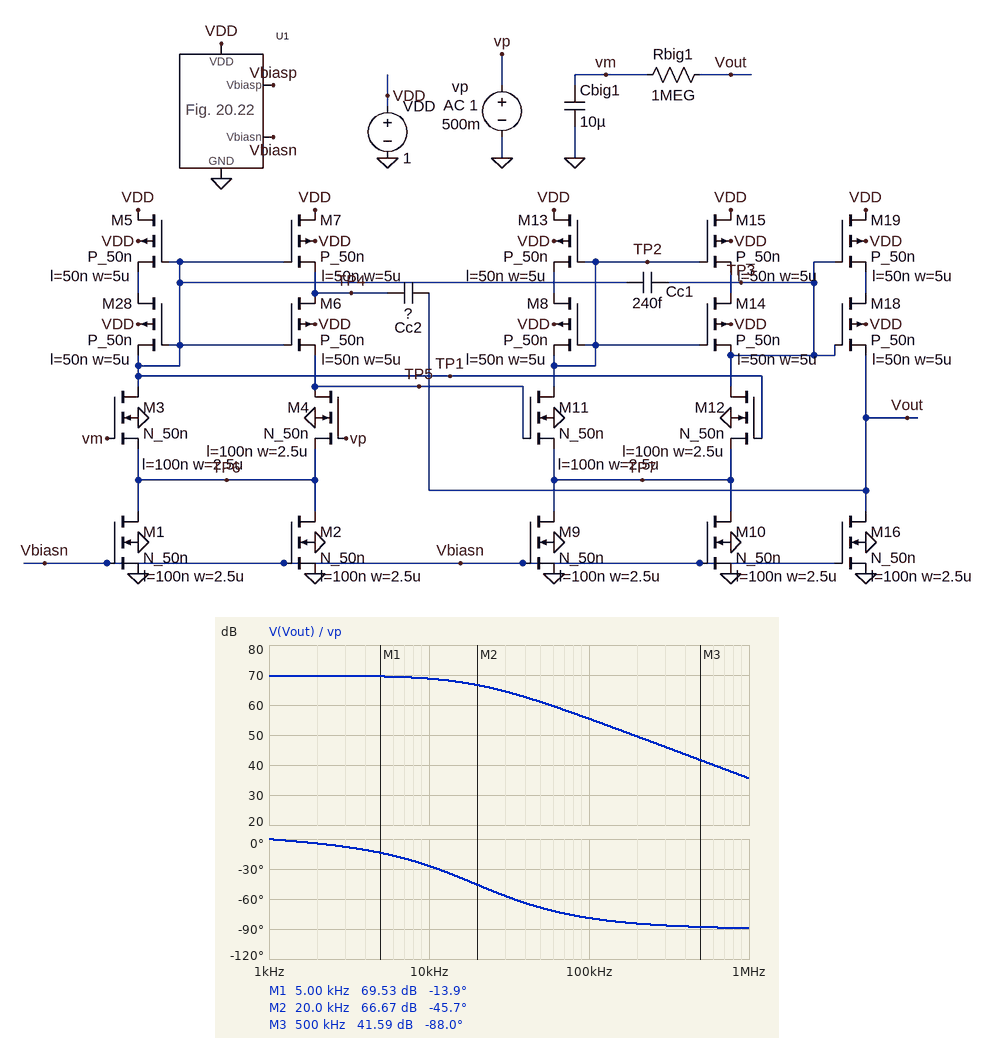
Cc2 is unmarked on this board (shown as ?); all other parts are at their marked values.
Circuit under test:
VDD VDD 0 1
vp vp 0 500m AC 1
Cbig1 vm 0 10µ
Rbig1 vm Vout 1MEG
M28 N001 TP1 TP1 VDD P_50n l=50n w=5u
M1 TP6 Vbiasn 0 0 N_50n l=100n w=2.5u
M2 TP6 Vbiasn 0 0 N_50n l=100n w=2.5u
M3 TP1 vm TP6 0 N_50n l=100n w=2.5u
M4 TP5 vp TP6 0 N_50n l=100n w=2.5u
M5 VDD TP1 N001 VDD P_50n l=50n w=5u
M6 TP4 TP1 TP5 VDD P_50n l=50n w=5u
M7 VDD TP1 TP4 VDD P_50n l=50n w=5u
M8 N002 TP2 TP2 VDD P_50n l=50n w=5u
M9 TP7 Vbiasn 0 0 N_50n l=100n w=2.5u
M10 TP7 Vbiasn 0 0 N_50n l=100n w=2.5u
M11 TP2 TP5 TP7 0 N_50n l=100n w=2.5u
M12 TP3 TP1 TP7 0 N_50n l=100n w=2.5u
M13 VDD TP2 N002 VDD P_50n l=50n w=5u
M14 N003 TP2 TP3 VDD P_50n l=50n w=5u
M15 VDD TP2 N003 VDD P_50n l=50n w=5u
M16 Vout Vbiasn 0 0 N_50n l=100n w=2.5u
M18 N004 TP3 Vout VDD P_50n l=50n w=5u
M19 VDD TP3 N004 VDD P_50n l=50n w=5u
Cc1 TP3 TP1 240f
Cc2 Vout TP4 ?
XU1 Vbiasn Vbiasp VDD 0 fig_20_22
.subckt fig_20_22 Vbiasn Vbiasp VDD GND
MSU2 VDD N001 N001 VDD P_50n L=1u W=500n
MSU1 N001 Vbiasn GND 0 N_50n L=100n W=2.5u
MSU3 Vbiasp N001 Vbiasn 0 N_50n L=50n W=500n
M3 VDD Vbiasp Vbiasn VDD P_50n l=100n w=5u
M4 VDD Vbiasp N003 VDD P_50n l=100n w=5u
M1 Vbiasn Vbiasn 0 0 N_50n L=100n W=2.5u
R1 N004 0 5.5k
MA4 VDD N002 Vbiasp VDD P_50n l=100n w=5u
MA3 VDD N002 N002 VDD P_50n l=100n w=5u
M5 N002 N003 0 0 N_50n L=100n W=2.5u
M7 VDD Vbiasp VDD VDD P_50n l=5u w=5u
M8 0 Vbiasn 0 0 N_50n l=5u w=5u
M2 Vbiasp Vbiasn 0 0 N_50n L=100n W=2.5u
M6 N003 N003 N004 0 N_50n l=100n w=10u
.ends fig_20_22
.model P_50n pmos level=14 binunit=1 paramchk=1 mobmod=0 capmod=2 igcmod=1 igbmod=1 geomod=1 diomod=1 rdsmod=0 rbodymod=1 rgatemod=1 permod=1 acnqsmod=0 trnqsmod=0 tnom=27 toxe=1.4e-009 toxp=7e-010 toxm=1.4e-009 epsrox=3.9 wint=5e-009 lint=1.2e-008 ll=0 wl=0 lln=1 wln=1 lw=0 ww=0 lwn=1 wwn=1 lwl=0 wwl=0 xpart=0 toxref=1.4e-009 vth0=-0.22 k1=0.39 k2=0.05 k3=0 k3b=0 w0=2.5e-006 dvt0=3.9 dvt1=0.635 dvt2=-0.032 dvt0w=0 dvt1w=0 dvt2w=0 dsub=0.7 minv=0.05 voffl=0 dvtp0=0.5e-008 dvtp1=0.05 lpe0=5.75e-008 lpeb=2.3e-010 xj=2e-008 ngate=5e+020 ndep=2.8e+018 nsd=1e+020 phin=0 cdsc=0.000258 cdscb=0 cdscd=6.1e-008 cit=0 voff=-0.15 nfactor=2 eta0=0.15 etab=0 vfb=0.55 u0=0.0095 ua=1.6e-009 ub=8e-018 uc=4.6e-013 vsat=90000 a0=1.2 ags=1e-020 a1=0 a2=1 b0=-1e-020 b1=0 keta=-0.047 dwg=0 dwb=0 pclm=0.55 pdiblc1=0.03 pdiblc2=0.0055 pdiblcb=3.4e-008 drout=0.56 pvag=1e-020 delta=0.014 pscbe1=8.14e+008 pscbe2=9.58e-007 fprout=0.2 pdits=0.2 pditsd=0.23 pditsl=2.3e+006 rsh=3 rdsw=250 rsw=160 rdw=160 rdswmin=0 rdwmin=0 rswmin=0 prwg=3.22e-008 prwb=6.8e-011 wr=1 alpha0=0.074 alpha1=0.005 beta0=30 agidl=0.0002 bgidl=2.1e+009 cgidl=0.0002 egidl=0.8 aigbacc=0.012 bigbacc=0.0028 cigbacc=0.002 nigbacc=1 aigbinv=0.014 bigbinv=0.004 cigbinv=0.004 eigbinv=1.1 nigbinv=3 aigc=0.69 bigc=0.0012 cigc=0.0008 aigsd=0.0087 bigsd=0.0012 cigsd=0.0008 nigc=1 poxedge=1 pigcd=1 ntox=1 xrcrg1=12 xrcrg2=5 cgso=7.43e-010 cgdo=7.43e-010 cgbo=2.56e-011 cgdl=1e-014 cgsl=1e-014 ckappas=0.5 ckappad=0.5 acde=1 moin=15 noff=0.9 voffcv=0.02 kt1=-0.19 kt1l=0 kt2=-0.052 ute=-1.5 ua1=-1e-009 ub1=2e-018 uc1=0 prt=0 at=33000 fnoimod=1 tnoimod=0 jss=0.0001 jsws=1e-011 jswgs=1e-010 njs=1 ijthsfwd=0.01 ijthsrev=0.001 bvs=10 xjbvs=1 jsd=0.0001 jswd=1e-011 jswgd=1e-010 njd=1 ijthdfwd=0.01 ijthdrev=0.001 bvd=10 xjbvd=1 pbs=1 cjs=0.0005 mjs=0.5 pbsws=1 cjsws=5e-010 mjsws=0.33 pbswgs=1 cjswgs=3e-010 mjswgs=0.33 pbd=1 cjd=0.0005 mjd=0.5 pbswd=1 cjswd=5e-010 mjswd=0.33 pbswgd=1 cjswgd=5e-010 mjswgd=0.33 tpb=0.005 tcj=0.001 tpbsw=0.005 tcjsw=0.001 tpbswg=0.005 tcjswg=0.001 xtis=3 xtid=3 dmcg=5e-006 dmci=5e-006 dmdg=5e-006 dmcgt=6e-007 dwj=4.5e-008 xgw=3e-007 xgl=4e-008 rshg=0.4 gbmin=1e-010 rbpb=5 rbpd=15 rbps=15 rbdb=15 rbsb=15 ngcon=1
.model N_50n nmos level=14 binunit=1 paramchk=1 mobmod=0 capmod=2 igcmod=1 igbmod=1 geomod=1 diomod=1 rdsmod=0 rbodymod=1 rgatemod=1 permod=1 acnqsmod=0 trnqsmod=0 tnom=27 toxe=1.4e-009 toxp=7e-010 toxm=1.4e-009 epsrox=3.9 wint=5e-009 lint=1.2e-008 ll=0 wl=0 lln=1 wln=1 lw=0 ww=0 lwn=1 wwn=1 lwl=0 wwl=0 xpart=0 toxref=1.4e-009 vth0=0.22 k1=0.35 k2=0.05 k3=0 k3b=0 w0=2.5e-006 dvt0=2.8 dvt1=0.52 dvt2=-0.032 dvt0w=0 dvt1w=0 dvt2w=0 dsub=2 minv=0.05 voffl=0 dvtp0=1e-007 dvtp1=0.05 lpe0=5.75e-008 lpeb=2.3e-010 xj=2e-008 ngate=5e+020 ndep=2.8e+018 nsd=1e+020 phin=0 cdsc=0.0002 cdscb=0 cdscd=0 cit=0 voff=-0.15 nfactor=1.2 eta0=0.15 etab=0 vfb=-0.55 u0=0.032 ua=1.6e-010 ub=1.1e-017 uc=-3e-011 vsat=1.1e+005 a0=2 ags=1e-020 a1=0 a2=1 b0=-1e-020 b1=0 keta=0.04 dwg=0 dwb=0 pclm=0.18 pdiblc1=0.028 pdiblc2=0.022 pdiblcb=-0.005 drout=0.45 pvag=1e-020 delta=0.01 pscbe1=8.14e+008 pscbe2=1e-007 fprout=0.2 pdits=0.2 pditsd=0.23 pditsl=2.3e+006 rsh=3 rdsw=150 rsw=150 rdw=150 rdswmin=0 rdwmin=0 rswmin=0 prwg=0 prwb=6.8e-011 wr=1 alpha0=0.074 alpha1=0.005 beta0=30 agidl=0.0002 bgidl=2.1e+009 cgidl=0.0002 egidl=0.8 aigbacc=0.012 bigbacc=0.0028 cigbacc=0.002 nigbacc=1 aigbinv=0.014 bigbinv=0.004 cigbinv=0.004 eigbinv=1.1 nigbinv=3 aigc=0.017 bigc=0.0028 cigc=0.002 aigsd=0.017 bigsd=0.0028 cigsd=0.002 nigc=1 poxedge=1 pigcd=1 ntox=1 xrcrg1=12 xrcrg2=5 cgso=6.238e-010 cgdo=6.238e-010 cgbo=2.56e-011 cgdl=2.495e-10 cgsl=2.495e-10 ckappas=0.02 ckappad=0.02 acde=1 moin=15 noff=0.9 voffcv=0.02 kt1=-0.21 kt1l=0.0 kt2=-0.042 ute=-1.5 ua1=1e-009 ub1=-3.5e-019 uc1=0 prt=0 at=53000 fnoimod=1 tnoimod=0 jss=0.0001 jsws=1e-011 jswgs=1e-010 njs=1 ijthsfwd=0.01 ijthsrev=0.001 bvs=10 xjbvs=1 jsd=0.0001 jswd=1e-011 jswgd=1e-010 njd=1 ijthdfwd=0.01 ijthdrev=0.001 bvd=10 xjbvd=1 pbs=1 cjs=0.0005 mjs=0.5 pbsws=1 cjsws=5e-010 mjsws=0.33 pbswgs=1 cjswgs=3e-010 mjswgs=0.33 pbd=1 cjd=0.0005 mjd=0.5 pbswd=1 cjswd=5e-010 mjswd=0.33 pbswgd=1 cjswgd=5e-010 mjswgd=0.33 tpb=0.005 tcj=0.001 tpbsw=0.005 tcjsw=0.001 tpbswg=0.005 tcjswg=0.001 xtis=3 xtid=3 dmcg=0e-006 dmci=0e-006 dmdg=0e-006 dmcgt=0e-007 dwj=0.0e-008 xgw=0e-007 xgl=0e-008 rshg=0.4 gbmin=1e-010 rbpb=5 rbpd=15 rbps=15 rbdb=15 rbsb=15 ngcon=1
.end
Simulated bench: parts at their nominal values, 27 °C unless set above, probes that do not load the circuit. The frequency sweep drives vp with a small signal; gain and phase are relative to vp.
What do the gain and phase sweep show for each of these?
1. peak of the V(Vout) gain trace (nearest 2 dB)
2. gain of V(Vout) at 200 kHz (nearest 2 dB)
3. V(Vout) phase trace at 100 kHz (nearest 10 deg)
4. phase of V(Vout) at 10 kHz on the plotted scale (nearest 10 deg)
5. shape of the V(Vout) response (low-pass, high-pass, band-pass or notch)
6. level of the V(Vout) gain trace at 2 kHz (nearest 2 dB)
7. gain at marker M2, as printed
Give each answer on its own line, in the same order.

70 dB
50 dB
-80 deg
-30 deg
low-pass
70 dB
66.67 dB
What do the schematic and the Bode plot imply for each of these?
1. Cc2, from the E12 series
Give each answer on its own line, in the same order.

680 fF
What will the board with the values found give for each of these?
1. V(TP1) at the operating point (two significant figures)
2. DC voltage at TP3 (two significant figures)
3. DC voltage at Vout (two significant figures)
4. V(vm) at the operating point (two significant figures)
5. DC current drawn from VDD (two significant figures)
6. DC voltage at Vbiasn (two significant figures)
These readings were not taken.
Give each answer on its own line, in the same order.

680 mV
670 mV
500 mV
500 mV
96 µA
350 mV
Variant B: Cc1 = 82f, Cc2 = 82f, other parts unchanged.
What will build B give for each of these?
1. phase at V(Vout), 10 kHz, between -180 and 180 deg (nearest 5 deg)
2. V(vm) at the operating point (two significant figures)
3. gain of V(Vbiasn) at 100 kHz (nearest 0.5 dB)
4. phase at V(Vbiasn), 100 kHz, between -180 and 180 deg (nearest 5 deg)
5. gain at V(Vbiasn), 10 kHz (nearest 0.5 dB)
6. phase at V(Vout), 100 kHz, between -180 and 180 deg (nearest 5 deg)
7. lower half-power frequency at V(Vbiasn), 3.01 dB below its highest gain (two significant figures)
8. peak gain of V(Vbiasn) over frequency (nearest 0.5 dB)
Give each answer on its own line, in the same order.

-5 deg
500 mV
-29.0 dB
50 deg
-45.5 dB
-35 deg
140 kHz
-24.0 dB
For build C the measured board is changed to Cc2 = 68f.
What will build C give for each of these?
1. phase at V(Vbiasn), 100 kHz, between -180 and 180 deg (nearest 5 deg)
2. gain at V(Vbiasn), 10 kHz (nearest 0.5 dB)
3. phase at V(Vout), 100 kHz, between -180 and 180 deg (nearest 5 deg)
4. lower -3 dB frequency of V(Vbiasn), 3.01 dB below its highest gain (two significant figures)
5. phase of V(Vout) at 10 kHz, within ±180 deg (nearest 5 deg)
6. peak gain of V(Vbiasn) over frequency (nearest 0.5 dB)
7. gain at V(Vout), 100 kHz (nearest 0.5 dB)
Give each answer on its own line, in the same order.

50 deg
-45.5 dB
-35 deg
140 kHz
-5 deg
-24.5 dB
68.0 dB
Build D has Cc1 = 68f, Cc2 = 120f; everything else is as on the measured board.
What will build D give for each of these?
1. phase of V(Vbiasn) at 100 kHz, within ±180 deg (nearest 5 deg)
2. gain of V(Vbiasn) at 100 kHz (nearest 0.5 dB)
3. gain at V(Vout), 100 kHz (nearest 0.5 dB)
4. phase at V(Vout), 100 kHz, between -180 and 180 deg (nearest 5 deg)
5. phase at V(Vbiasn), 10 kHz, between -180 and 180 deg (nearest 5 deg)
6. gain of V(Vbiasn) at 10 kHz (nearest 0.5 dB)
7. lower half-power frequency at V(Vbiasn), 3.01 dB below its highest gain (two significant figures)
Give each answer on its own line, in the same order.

40 deg
-30.0 dB
67.0 dB
-45 deg
45 deg
-45.5 dB
100 kHz
